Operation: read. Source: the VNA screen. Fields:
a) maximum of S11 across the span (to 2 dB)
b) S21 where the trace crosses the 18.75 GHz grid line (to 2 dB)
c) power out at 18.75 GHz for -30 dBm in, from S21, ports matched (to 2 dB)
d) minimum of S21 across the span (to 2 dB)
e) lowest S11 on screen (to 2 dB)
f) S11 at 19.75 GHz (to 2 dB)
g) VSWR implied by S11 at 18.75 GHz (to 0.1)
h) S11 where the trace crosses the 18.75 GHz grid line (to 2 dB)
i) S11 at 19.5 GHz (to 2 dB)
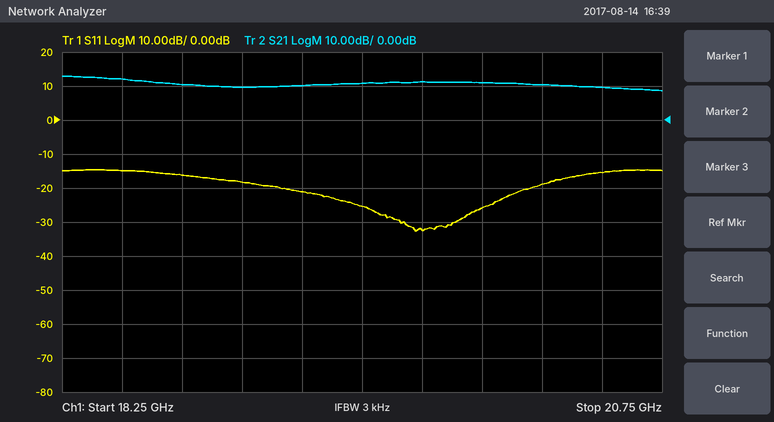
-14 dB
10 dB
-20 dBm
8 dB
-32 dB
-32 dB
1.4
-16 dB
-26 dB
